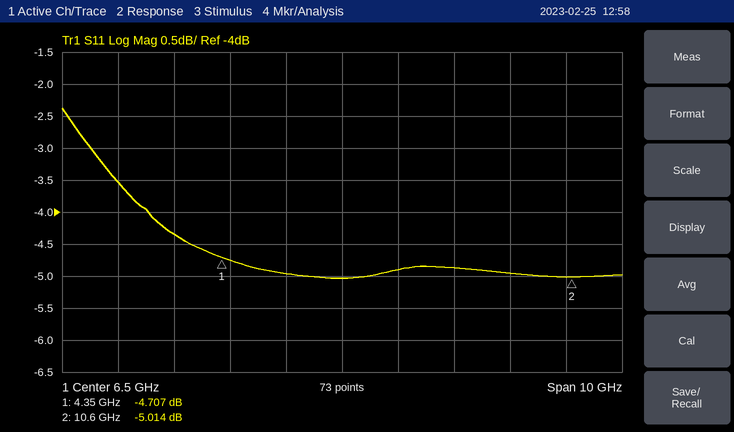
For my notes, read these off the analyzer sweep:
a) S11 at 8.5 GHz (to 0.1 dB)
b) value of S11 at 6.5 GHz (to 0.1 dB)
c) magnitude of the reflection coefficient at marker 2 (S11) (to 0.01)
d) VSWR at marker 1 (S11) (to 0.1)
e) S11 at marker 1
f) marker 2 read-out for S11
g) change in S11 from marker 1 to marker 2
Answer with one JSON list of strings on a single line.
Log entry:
["-4.9 dB", "-5.0 dB", "0.56", "3.8", "-4.707 dB", "-5.014 dB", "-0.307 dB"]
